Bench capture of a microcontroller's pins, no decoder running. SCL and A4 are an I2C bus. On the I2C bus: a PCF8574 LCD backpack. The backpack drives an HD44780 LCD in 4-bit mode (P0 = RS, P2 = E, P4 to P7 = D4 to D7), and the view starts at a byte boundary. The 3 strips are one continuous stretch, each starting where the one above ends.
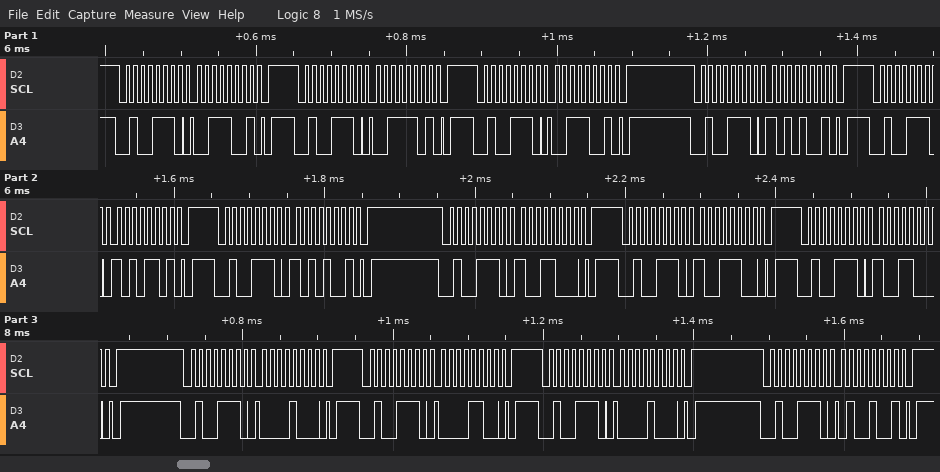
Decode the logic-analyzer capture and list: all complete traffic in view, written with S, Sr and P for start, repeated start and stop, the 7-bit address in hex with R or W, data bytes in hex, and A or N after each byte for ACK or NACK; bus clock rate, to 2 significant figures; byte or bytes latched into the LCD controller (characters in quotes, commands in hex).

S 27W A 39 A P S 27W A 3D A P S 27W A 39 A P S 27W A A9 A P S 27W A AD A P S 27W A A9 A P S 27W A 98 A P S 27W A 9C A P S 27W A 98 A P S 27W A 08 A P S 27W A 0C A P S 27W A 08 A P S 27W A 49 A P
100 kHz
':' 0x90
